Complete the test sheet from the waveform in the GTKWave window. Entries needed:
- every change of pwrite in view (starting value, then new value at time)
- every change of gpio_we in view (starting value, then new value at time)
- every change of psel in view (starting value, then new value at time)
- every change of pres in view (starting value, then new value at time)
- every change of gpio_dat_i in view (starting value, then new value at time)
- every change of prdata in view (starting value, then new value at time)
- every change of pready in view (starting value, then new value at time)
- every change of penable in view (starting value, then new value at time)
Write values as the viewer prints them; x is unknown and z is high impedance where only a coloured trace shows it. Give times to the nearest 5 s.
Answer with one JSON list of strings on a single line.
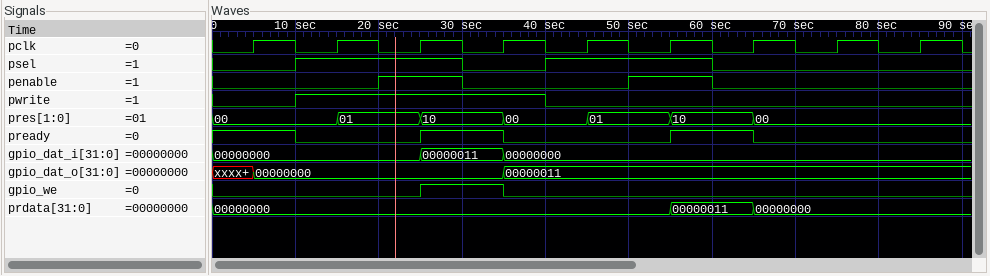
["0, 1 at 10 s, 0 at 40 s", "0, 1 at 25 s, 0 at 35 s", "0, 1 at 10 s, 0 at 30 s, 1 at 40 s, 0 at 60 s", "00, 01 at 15 s, 10 at 25 s, 00 at 35 s, 01 at 45 s, 10 at 55 s, 00 at 65 s", "00000000, 00000011 at 25 s, 00000000 at 35 s", "00000000, 00000011 at 55 s, 00000000 at 65 s", "1, 0 at 10 s, 1 at 25 s, 0 at 35 s, 1 at 55 s, 0 at 65 s", "0, 1 at 20 s, 0 at 30 s, 1 at 50 s, 0 at 60 s"]
